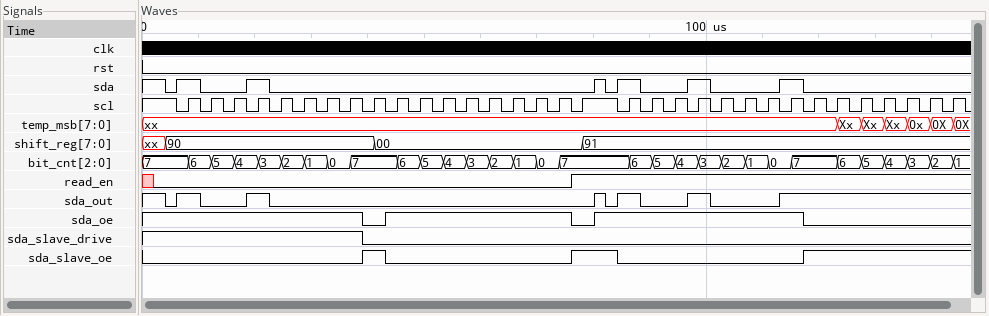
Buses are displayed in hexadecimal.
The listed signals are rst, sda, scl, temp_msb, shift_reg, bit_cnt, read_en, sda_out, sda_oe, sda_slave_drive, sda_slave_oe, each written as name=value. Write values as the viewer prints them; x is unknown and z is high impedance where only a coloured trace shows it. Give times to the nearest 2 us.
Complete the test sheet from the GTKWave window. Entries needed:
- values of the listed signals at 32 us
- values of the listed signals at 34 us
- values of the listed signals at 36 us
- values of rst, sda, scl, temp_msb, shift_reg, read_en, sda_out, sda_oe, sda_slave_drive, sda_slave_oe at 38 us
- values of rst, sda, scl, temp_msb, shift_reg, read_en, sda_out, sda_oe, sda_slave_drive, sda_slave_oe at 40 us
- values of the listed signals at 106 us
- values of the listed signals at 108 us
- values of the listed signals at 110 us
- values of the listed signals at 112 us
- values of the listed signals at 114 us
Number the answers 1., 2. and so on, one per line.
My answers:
1. rst=0, sda=0, scl=0, temp_msb=xx, shift_reg=90, bit_cnt=1, read_en=0, sda_out=0, sda_oe=1, sda_slave_drive=1, sda_slave_oe=0
2. rst=0, sda=0, scl=1, temp_msb=xx, shift_reg=90, bit_cnt=0, read_en=0, sda_out=0, sda_oe=1, sda_slave_drive=1, sda_slave_oe=0
3. rst=0, sda=0, scl=0, temp_msb=xx, shift_reg=90, bit_cnt=0, read_en=0, sda_out=0, sda_oe=1, sda_slave_drive=1, sda_slave_oe=0
4. rst=0, sda=0, scl=1, temp_msb=xx, shift_reg=90, read_en=0, sda_out=0, sda_oe=1, sda_slave_drive=1, sda_slave_oe=0
5. rst=0, sda=0, scl=0, temp_msb=xx, shift_reg=90, read_en=0, sda_out=0, sda_oe=0, sda_slave_drive=0, sda_slave_oe=1
6. rst=0, sda=0, scl=0, temp_msb=xx, shift_reg=91, bit_cnt=2, read_en=1, sda_out=0, sda_oe=1, sda_slave_drive=0, sda_slave_oe=0
7. rst=0, sda=0, scl=1, temp_msb=xx, shift_reg=91, bit_cnt=1, read_en=1, sda_out=0, sda_oe=1, sda_slave_drive=0, sda_slave_oe=0
8. rst=0, sda=0, scl=0, temp_msb=xx, shift_reg=91, bit_cnt=1, read_en=1, sda_out=0, sda_oe=1, sda_slave_drive=0, sda_slave_oe=0
9. rst=0, sda=0, scl=1, temp_msb=xx, shift_reg=91, bit_cnt=0, read_en=1, sda_out=0, sda_oe=1, sda_slave_drive=0, sda_slave_oe=0
10. rst=0, sda=1, scl=0, temp_msb=xx, shift_reg=91, bit_cnt=0, read_en=1, sda_out=1, sda_oe=1, sda_slave_drive=0, sda_slave_oe=0
